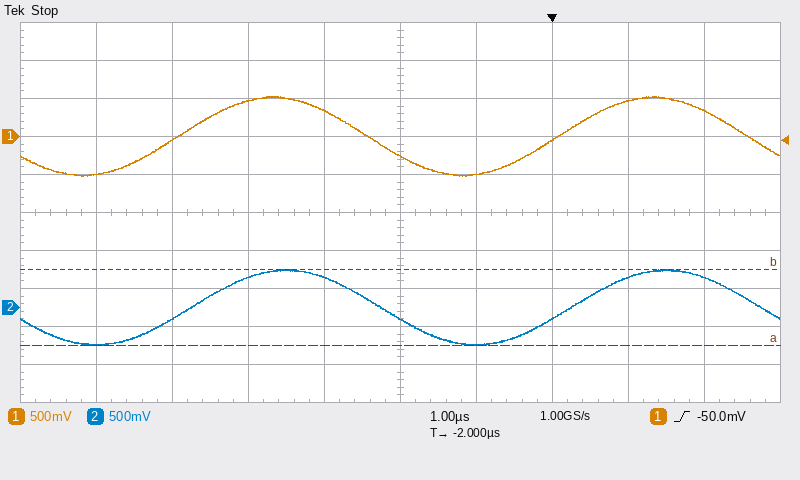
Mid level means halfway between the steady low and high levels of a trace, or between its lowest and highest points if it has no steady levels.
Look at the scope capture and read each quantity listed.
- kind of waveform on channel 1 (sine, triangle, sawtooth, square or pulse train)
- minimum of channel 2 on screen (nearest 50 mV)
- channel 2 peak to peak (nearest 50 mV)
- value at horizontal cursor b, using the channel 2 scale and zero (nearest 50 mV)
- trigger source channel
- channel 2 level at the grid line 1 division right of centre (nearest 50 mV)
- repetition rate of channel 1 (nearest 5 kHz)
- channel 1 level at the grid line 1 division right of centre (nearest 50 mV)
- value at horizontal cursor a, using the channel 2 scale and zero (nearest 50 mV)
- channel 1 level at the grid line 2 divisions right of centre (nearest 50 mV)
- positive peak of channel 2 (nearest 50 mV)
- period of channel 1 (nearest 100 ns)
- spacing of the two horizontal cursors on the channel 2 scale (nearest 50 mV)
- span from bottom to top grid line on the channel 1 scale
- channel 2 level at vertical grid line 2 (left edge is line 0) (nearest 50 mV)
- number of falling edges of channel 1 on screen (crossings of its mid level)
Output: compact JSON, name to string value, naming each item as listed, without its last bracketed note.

{"kind of waveform on channel 1": "sine", "minimum of channel 2 on screen": "-500 mV", "channel 2 peak to peak": "1.00 V", "value at horizontal cursor b, using the channel 2 scale and zero": "500 mV", "trigger source channel": "channel 1", "channel 2 level at the grid line 1 division right of centre": "-500 mV", "repetition rate of channel 1": "200 kHz", "channel 1 level at the grid line 1 division right of centre": "-500 mV", "value at horizontal cursor a, using the channel 2 scale and zero": "-500 mV", "channel 1 level at the grid line 2 divisions right of centre": "-50 mV", "positive peak of channel 2": "500 mV", "period of channel 1": "5.0 µs", "spacing of the two horizontal cursors on the channel 2 scale": "1.00 V", "span from bottom to top grid line on the channel 1 scale": "5 V", "channel 2 level at vertical grid line 2 (left edge is line 0)": "-150 mV", "number of falling edges of channel 1 on screen": "2"}
